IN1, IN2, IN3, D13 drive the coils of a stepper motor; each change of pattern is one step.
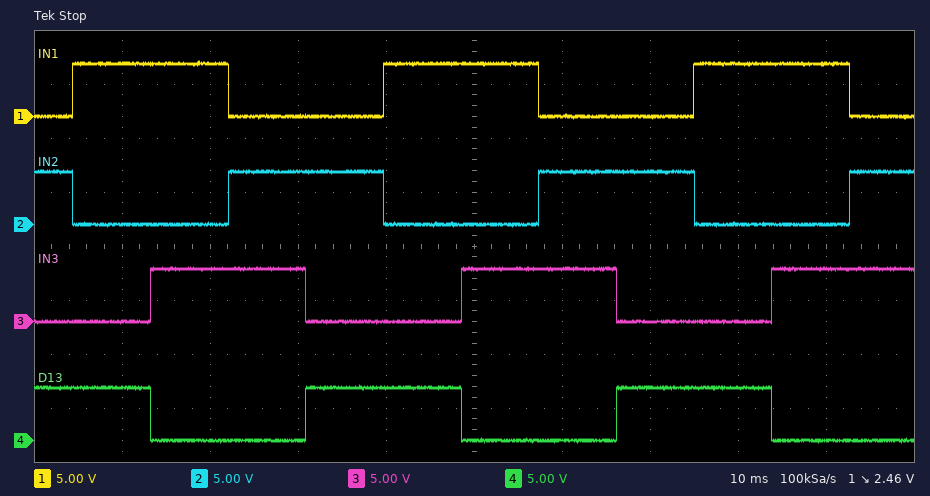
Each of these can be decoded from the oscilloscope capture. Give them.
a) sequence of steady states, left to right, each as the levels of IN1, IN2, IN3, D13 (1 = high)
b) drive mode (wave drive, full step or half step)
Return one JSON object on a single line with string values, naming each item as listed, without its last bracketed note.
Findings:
{"sequence of steady states, left to right, each as the levels of IN1, IN2, IN3, D13": "0101 1001 1010 0110 0101 1001 1010 0110 0101 1001 1010 0110", "drive mode": "full step"}
